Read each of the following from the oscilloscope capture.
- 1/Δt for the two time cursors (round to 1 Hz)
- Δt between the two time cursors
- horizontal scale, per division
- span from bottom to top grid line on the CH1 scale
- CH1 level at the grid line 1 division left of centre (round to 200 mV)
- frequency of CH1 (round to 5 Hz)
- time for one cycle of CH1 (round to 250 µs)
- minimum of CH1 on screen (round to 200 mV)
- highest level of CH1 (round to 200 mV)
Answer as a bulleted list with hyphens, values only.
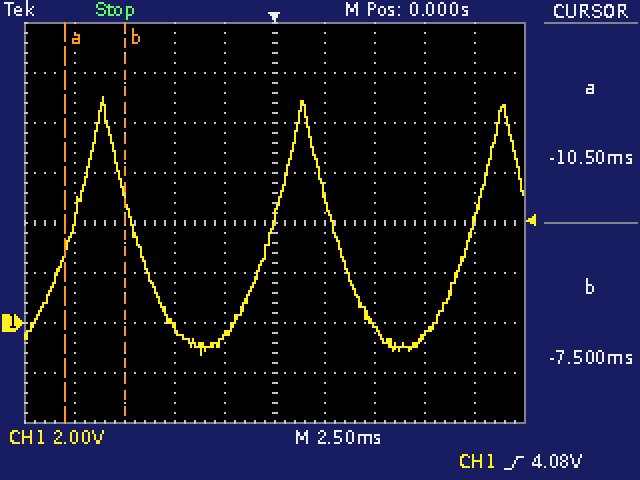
- 333 Hz
- 3.00 ms
- 2.5 ms
- 16 V
- -400 mV
- 100 Hz
- 10.00 ms
- -1.2 V
- 9.0 V
